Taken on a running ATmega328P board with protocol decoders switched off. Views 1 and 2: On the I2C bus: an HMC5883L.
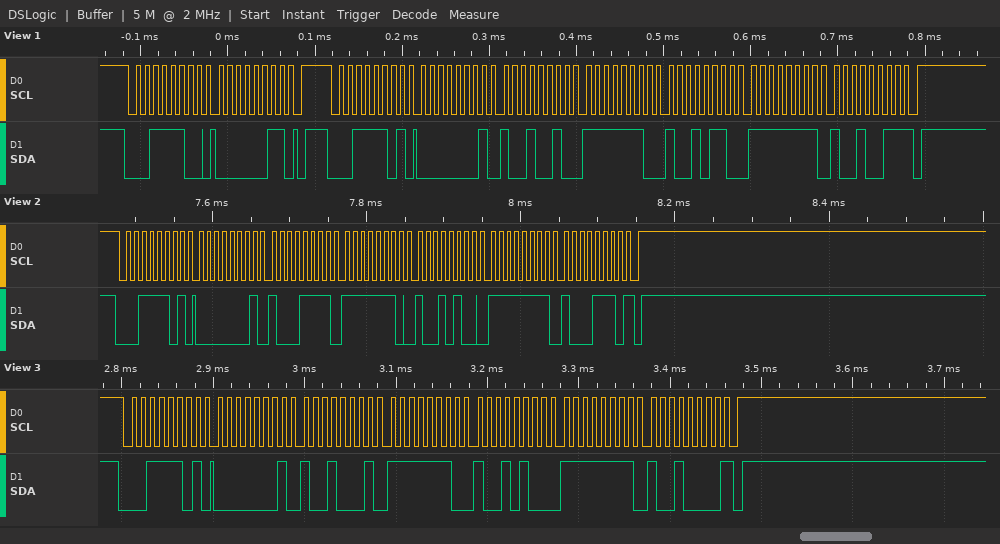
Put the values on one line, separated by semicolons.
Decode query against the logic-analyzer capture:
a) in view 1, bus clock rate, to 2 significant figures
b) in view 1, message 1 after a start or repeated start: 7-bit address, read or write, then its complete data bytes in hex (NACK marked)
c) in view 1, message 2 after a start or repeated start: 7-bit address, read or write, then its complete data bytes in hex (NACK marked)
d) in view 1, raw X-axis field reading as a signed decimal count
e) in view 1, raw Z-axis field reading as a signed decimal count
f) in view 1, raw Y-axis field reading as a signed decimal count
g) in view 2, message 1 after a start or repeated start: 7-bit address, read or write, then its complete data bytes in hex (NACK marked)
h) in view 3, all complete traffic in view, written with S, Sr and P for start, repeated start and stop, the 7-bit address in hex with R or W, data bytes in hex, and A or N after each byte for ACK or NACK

100 kHz; 0x1E write: 03; 0x1E read: 01 92 FE 96 FF 93 NACK; 402; -362; -109; 0x1E read: 01 8F FE 94 FF 8E NACK; S 1ER A 01 A 91 A FE A 94 A FF A 90 N P
